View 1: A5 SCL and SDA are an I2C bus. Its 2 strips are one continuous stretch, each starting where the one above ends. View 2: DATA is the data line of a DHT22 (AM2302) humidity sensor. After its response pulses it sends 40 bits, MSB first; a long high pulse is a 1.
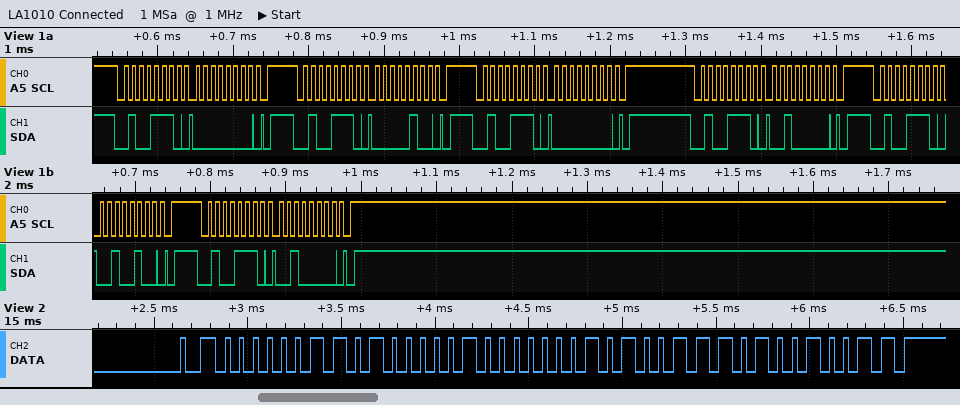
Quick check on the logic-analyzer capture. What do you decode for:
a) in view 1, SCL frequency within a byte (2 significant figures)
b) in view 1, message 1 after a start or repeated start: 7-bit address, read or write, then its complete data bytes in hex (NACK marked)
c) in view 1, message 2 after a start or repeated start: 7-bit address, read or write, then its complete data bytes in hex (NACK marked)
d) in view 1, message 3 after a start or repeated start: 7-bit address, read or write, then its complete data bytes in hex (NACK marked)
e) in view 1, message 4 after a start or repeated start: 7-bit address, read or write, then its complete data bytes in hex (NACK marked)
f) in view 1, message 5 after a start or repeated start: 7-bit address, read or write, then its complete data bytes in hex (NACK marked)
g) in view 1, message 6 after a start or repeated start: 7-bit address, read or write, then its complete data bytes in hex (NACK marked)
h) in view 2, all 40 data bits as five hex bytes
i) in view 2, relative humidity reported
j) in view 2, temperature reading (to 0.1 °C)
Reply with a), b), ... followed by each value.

a) 100 kHz
b) 0x27 write: 00
c) 0x27 write: 04
d) 0x27 write: 00
e) 0x27 write: 20
f) 0x27 write: 24
g) 0x27 write: 20
h) 03 41 01 4E 93
i) 83.3 %
j) 33.4 °C
